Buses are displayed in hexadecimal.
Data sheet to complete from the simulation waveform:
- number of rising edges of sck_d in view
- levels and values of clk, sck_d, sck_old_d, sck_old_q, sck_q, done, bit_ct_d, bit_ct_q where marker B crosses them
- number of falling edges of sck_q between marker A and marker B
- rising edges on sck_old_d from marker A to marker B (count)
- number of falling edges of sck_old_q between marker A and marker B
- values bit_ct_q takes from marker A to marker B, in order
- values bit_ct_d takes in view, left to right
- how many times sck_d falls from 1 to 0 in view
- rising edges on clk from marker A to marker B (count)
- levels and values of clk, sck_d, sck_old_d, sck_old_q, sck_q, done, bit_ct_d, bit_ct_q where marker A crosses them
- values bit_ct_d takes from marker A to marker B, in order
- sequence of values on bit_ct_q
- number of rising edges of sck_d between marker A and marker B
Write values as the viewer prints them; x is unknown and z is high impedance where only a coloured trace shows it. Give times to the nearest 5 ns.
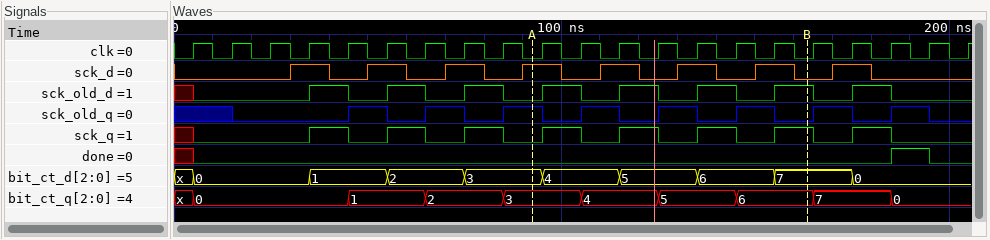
8
clk=0, sck_d=0, sck_old_d=1, sck_old_q=0, sck_q=1, done=0, bit_ct_d=7, bit_ct_q=6
3
4
4
3, 4, 5, 6
x, 0, 1, 2, 3, 4, 5, 6, 7, 0
8
7
clk=0, sck_d=1, sck_old_d=0, sck_old_q=1, sck_q=0, done=0, bit_ct_d=3, bit_ct_q=3
3, 4, 5, 6, 7
x, 0, 1, 2, 3, 4, 5, 6, 7, 0
3
